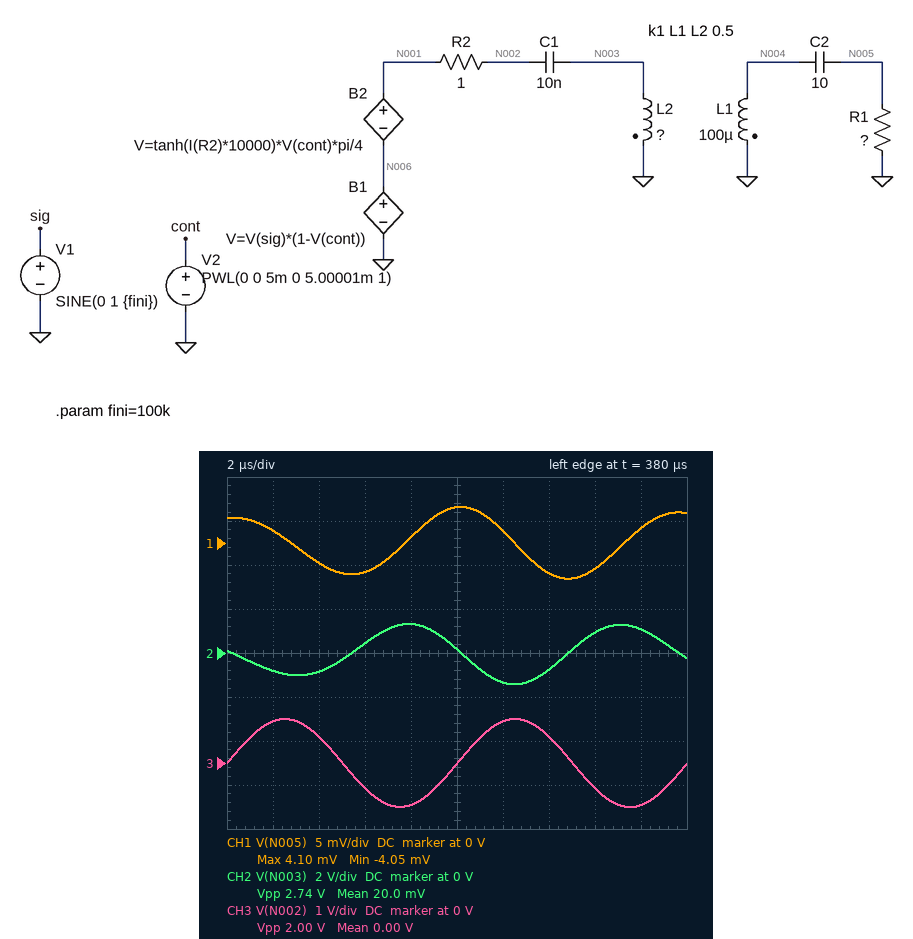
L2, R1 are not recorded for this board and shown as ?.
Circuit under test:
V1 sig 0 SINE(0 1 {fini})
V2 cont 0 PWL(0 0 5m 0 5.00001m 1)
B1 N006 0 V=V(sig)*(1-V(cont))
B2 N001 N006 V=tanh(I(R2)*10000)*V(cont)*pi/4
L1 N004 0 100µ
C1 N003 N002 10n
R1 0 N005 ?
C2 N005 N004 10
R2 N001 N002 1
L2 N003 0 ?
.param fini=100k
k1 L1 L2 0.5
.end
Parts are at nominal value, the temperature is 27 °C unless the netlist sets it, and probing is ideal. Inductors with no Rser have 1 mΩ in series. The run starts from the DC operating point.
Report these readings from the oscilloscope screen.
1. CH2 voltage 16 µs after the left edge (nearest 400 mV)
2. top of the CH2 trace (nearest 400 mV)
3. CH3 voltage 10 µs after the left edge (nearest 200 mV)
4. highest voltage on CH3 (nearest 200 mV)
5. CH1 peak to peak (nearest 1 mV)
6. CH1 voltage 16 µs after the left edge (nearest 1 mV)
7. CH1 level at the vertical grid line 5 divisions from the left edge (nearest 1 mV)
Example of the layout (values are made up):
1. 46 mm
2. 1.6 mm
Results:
1. 800 mV
2. 1.2 V
3. 0 V
4. 1.0 V
5. 8 mV
6. -3 mV
7. 4 mV
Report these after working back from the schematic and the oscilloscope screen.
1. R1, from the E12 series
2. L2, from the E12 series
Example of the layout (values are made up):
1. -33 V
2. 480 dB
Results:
1. 0.39 Ω
2. 180 µH
